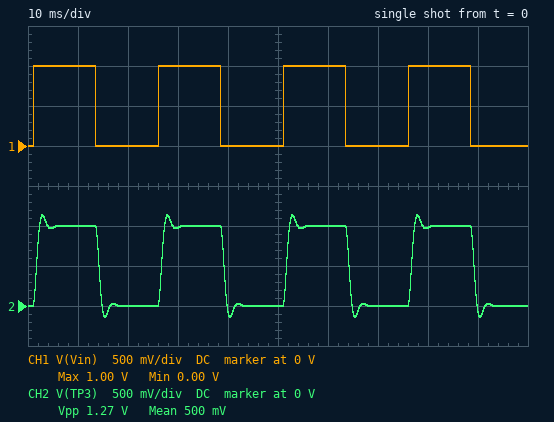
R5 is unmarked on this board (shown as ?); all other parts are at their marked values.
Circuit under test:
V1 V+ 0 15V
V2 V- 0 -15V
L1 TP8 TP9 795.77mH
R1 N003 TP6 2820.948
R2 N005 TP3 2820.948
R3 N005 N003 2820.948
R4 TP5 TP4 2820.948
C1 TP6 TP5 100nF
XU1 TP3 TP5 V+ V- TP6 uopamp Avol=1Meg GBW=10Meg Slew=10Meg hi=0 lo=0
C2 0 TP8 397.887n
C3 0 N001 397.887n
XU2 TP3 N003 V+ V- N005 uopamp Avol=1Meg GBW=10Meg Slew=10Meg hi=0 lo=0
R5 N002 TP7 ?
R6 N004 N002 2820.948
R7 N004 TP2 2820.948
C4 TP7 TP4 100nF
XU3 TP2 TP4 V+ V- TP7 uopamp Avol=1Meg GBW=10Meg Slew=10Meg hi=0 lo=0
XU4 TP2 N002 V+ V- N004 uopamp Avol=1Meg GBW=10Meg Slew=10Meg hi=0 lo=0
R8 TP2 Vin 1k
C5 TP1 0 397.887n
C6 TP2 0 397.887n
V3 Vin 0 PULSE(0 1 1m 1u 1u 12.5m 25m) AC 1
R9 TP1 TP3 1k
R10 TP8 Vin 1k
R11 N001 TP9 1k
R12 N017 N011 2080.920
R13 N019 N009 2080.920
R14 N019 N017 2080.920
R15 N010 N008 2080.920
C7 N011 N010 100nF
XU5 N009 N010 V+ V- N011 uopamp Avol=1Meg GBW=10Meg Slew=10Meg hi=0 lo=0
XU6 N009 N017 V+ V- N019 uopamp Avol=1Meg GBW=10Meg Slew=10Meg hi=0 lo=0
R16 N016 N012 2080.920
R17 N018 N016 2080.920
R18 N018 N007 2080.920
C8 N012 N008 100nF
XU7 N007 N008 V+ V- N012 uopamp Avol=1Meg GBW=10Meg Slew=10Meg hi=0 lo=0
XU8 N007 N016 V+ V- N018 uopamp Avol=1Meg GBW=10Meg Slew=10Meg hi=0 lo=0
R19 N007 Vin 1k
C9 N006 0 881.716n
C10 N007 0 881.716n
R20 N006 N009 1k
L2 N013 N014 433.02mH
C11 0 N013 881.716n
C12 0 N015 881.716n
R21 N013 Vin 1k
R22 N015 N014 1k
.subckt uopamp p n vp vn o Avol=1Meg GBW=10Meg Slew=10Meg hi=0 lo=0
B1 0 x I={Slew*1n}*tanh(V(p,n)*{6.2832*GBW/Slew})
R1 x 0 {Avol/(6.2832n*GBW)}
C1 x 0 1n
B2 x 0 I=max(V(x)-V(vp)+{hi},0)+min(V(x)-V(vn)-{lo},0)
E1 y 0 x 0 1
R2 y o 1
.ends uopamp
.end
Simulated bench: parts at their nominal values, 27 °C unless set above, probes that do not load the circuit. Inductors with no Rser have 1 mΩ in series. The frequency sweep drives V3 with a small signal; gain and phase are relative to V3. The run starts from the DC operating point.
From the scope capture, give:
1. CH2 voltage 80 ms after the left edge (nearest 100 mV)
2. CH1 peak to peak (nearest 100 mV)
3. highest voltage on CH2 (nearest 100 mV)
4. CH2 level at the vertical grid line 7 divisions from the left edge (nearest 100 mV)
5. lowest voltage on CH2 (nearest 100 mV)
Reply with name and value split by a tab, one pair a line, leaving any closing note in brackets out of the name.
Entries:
CH2 voltage 80 ms after the left edge	1.0 V
CH1 peak to peak	1.0 V
highest voltage on CH2	1.1 V
CH2 level at the vertical grid line 7 divisions from the left edge	0 V
lowest voltage on CH2	-100 mV
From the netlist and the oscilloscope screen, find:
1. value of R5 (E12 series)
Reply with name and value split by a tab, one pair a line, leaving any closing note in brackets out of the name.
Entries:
value of R5	5.6 kΩ
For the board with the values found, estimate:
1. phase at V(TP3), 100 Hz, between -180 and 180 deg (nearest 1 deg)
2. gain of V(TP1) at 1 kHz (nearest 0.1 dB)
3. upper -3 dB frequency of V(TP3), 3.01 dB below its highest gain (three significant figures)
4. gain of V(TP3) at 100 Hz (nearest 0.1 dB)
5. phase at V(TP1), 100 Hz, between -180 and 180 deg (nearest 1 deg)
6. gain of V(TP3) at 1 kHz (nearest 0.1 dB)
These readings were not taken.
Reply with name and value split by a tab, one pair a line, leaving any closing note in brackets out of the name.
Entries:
phase at V(TP3), 100 Hz, between -180 and 180 deg	-22 deg
gain of V(TP1) at 1 kHz	-29.7 dB
upper -3 dB frequency of V(TP3), 3.01 dB below its highest gain	375 Hz
gain of V(TP3) at 100 Hz	0.2 dB
phase at V(TP1), 100 Hz, between -180 and 180 deg	-36 deg
gain of V(TP3) at 1 kHz	-21.1 dB
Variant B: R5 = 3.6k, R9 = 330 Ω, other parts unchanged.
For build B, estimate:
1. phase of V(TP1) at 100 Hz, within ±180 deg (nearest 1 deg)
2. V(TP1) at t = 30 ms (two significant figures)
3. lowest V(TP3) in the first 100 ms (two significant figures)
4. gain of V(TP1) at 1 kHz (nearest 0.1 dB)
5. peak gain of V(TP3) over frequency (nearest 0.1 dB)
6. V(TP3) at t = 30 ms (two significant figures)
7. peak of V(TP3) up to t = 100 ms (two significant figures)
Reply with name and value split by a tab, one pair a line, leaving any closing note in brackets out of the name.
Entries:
phase of V(TP1) at 100 Hz, within ±180 deg	-30 deg
V(TP1) at t = 30 ms	940 mV
lowest V(TP3) in the first 100 ms	-200 mV
gain of V(TP1) at 1 kHz	-29.3 dB
peak gain of V(TP3) over frequency	2.2 dB
V(TP3) at t = 30 ms	960 mV
peak of V(TP3) up to t = 100 ms	1.2 V
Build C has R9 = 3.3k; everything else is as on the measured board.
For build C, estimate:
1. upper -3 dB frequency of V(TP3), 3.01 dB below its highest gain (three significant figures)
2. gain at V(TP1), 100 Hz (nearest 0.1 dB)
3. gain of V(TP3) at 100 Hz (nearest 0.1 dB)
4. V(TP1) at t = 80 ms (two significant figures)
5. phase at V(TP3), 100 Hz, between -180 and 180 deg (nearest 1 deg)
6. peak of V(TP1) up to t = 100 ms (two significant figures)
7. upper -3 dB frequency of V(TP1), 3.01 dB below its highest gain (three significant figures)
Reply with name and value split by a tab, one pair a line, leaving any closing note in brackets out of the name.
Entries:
upper -3 dB frequency of V(TP3), 3.01 dB below its highest gain	369 Hz
gain at V(TP1), 100 Hz	-2.6 dB
gain of V(TP3) at 100 Hz	-0.3 dB
V(TP1) at t = 80 ms	920 mV
phase at V(TP3), 100 Hz, between -180 and 180 deg	-21 deg
peak of V(TP1) up to t = 100 ms	1.0 V
upper -3 dB frequency of V(TP1), 3.01 dB below its highest gain	110 Hz
